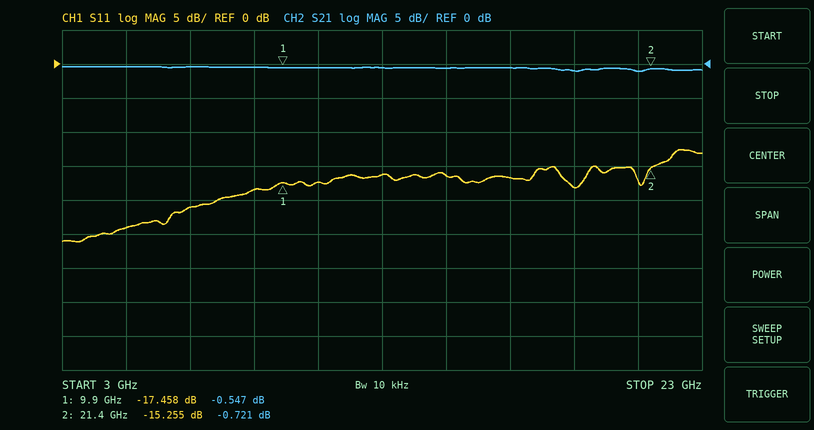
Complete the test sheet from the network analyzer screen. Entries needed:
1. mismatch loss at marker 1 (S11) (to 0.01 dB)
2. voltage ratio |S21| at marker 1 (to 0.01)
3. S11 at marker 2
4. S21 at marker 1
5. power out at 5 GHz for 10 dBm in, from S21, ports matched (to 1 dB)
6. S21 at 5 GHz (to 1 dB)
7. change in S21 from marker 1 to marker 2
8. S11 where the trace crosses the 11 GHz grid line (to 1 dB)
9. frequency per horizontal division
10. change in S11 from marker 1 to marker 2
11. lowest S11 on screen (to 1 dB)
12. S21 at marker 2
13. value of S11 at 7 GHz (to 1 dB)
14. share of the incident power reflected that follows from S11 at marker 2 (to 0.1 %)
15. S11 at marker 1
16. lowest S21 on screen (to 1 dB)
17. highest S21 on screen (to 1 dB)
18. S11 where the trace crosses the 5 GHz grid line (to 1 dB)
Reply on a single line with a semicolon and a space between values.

0.08 dB; 0.94; -15.255 dB; -0.547 dB; 10 dBm; 0 dB; -0.174 dB; -17 dB; 2 GHz; 2.203 dB; -26 dB; -0.721 dB; -21 dB; 3.0 %; -17.458 dB; -1 dB; 0 dB; -24 dB
